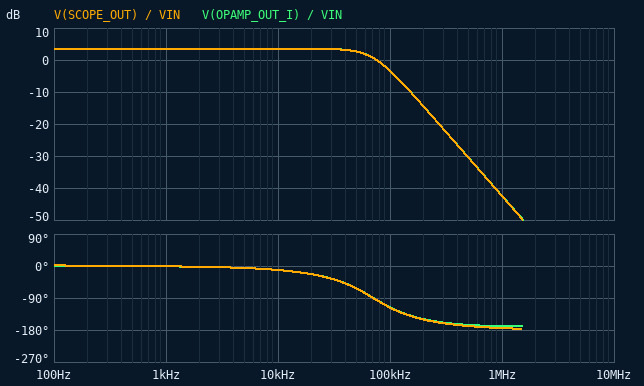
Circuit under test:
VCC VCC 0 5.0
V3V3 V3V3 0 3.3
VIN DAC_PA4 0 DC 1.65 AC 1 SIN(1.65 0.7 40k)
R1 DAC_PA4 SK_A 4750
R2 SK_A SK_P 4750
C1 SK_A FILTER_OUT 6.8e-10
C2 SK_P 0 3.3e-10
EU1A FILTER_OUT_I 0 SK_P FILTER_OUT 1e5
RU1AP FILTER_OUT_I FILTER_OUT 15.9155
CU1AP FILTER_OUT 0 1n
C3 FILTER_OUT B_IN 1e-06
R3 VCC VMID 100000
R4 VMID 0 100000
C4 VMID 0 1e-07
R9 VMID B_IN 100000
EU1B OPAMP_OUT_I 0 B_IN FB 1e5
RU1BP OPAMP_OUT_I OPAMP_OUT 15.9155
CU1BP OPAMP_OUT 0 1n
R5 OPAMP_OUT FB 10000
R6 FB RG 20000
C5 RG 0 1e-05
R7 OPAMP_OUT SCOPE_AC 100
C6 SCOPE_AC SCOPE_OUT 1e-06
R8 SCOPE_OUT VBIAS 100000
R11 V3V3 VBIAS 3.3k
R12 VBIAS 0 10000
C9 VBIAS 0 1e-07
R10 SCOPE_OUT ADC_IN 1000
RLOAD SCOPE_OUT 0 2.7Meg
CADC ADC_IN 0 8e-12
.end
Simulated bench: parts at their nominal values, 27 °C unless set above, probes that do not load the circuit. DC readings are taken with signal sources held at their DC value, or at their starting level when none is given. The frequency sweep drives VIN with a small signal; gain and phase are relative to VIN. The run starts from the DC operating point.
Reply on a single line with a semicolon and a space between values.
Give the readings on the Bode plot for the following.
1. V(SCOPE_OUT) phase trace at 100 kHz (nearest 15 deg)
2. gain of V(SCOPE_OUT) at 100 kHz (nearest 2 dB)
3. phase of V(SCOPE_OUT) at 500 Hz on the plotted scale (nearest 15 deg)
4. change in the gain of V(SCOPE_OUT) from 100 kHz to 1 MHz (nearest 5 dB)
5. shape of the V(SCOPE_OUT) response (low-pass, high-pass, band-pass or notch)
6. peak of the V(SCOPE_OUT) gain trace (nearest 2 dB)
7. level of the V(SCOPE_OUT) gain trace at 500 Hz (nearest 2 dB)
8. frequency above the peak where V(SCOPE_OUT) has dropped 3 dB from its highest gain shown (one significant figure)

-120 deg; -4 dB; 0 deg; -40 dB; low-pass; 4 dB; 4 dB; 70 kHz
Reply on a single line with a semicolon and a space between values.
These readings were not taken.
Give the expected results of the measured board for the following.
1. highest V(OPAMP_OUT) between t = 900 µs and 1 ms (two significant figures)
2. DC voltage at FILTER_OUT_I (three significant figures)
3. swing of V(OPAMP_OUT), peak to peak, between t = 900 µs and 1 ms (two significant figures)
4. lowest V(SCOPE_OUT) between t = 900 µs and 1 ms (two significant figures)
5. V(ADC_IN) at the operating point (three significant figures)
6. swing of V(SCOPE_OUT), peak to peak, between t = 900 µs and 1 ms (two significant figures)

3.5 V; 1.65 V; 2.0 V; 1.4 V; 2.39 V; 2.0 V
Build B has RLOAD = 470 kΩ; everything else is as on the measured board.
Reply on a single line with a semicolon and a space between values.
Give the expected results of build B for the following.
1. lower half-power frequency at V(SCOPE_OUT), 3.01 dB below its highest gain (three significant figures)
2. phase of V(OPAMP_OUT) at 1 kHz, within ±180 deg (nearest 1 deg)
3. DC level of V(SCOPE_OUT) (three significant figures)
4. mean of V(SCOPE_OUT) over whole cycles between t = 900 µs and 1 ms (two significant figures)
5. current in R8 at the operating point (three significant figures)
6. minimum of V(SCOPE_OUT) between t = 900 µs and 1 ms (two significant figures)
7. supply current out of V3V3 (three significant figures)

2.49 Hz; -1 deg; 2.04 V; 2.0 V; 4.33 µA; 1.0 V; 251 µA
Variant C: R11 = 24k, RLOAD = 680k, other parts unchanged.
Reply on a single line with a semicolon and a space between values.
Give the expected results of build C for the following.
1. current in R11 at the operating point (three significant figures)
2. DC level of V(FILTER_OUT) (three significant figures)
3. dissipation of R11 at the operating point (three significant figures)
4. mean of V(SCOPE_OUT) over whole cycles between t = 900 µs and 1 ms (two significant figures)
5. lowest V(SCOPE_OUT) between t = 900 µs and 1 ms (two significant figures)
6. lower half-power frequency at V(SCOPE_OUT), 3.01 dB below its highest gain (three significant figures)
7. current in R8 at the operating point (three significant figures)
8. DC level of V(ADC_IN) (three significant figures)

97.4 µA; 1.65 V; 228 µW; 840 mV; -170 mV; 2.35 Hz; 1.23 µA; 839 mV
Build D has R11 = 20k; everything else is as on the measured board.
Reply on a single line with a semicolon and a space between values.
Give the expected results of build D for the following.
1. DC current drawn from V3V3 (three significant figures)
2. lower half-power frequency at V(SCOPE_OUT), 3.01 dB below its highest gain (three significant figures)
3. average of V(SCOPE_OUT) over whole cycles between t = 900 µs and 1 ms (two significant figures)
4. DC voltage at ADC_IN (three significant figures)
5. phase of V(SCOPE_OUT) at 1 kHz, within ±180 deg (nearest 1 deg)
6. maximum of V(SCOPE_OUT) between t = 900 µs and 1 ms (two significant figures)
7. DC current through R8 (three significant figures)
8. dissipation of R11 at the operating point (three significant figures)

110 µA; 2.21 Hz; 1.1 V; 1.06 V; -1 deg; 2.1 V; 392 nA; 243 µW
